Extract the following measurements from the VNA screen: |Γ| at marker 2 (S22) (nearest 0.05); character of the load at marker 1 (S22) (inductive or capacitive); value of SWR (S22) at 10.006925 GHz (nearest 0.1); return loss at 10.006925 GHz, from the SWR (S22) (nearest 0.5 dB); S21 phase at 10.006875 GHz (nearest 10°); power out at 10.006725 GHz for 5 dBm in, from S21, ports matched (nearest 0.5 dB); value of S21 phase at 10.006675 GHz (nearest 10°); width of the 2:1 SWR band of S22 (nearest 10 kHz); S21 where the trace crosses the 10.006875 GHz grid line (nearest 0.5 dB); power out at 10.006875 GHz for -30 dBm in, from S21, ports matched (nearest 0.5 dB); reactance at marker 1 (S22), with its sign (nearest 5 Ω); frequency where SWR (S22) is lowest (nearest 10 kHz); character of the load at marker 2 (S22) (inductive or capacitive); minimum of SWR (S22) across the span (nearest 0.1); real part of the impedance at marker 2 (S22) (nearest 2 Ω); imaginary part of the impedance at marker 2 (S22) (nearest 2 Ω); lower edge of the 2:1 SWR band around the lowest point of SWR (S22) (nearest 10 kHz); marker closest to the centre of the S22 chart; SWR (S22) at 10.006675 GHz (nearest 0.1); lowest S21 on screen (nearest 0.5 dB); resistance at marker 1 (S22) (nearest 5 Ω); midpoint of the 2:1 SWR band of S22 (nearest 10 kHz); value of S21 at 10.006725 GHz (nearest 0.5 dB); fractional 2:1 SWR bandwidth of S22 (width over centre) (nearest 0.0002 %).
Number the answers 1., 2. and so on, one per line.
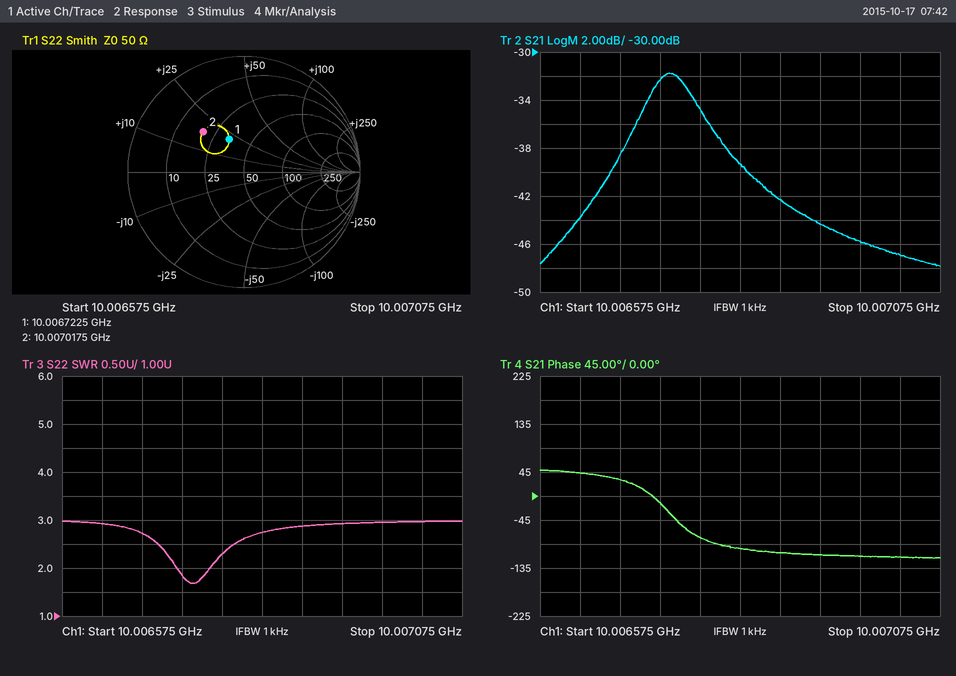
1. 0.50
2. inductive
3. 2.9
4. 6.0 dB
5. -110°
6. -27.5 dBm
7. 30°
8. 40 kHz
9. -42.5 dB
10. -72.5 dBm
11. +20 Ω
12. 10.00674 GHz
13. inductive
14. 1.7
15. 20 Ω
16. +18 Ω
17. 10.00672 GHz
18. marker 1
19. 2.7
20. -48.0 dB
21. 35 Ω
22. 10.00674 GHz
23. -32.5 dB
24. 0.0004 %
